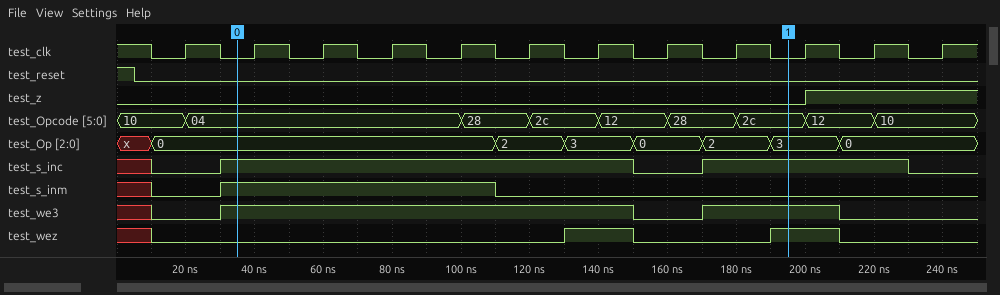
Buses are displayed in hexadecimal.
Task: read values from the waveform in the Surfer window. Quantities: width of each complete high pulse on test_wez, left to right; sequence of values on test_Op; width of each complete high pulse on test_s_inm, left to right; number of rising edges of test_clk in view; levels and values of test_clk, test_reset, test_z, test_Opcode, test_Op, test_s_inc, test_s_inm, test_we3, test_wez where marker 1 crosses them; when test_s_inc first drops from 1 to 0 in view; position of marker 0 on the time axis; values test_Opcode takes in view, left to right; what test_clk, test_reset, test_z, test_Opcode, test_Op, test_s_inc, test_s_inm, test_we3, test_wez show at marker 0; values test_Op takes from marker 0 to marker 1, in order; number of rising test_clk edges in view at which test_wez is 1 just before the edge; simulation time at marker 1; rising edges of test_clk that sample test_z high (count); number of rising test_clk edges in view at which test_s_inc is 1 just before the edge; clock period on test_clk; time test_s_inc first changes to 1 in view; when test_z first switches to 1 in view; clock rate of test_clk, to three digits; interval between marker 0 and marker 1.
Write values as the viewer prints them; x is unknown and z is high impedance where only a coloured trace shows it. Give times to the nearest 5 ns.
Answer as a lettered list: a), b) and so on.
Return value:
a) 20 ns, 20 ns
b) x, 0, 2, 3, 0, 2, 3, 0
c) 80 ns
d) 12
e) test_clk=0, test_reset=0, test_z=0, test_Opcode=2c, test_Op=3, test_s_inc=1, test_s_inm=0, test_we3=1, test_wez=1
f) 150 ns
g) 35 ns
h) 10, 04, 28, 2c, 12, 28, 2c, 12, 10
i) test_clk=0, test_reset=0, test_z=0, test_Opcode=04, test_Op=0, test_s_inc=1, test_s_inm=1, test_we3=1, test_wez=0
j) 0, 2, 3, 0, 2, 3
k) 2
l) 195 ns
m) 2
n) 9
o) 20 ns
p) 30 ns
q) 200 ns
r) 50.0 MHz
s) 160 ns
